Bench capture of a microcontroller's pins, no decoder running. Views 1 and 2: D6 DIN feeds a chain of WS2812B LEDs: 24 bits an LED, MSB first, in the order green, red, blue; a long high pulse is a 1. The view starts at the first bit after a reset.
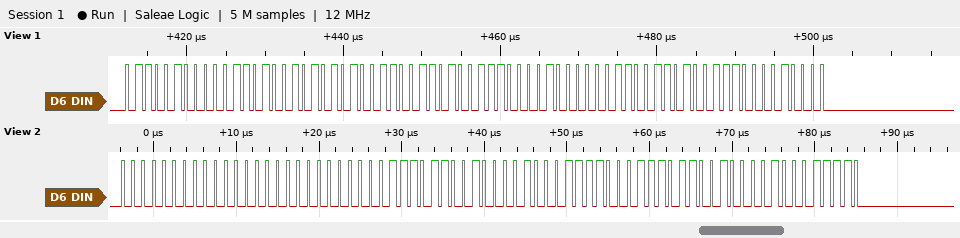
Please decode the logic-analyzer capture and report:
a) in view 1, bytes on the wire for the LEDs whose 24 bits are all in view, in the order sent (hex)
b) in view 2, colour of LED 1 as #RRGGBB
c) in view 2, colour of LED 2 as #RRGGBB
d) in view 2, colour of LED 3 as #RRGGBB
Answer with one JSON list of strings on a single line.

["64 1A 55 33 4E 10 33 4E 10", "#000000", "#213B1E", "#213B1E"]
